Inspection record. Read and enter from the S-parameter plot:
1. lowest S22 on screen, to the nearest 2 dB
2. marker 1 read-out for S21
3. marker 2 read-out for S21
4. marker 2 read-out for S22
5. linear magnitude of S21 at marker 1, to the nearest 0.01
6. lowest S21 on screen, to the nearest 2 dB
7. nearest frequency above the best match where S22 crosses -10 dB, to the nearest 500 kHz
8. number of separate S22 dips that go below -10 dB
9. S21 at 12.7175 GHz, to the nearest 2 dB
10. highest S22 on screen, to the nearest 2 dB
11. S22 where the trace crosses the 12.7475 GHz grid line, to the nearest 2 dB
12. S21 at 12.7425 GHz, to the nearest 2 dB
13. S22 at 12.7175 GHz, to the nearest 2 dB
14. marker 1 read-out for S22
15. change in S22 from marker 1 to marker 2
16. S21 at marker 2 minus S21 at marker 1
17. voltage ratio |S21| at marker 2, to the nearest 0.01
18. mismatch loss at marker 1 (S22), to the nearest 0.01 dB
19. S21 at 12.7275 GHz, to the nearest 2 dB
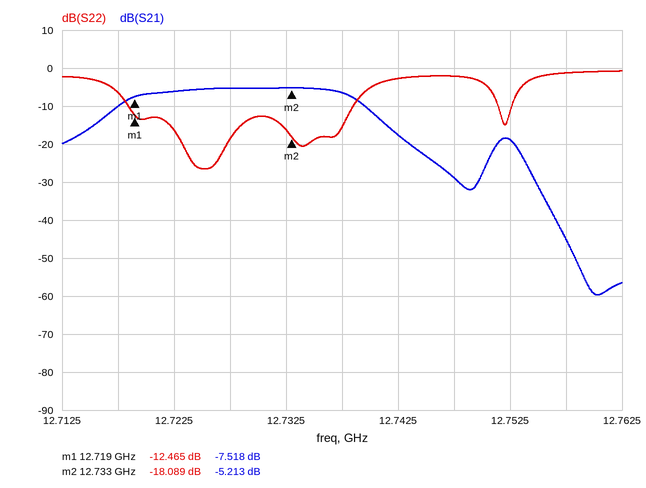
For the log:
-26 dB
-7.518 dB
-5.213 dB
-18.089 dB
0.42
-60 dB
12.7385 GHz
3
-10 dB
0 dB
-2 dB
-18 dB
-6 dB
-12.465 dB
-5.624 dB
2.305 dB
0.55
0.25 dB
-6 dB
